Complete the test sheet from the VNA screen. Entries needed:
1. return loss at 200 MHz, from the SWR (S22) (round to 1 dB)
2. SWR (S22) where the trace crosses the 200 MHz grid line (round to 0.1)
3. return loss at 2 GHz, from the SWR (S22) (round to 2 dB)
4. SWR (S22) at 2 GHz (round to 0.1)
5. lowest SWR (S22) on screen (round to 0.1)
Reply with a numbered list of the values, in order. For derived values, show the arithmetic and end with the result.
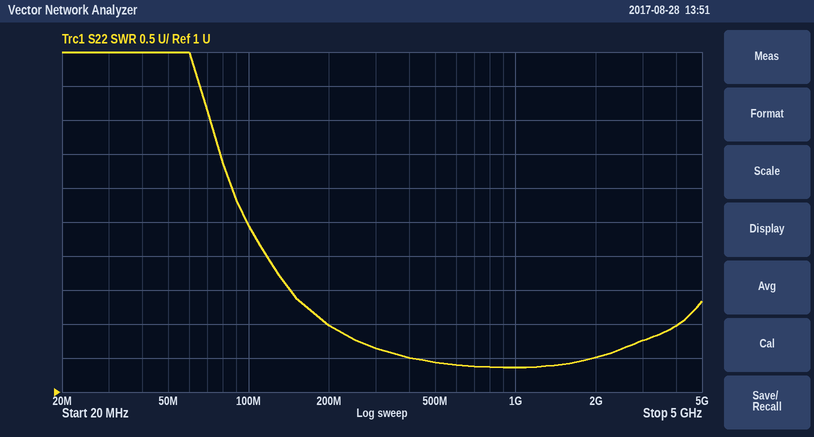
1. −20 log10((2 − 1)/(2 + 1)) ≈ 10 dB
2. 2.0
3. −20 log10((1.5 − 1)/(1.5 + 1)) ≈ 14 dB
4. 1.5
5. 1.4
